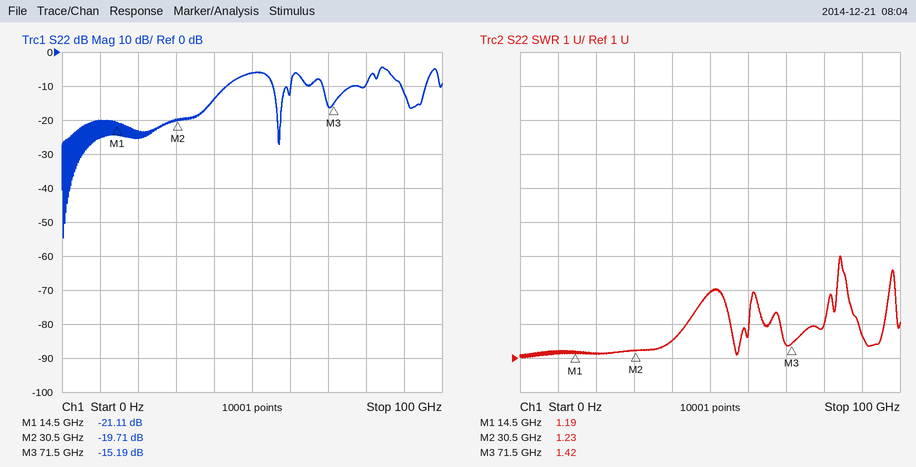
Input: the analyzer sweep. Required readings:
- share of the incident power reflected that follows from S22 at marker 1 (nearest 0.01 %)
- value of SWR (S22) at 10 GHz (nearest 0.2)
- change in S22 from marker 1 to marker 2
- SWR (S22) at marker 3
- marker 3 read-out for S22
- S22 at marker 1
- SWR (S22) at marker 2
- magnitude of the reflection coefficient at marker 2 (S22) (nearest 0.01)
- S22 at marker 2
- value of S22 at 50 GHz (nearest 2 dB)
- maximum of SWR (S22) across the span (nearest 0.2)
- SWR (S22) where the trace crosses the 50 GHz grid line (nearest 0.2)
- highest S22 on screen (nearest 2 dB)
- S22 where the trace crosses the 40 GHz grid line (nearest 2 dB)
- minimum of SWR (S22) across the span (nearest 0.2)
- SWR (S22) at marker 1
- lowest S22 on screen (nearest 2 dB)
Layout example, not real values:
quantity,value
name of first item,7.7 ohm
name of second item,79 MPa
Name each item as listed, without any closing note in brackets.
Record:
quantity,value
share of the incident power reflected that follows from S22 at marker 1,0.77 %
value of SWR (S22) at 10 GHz,1.2
change in S22 from marker 1 to marker 2,1.40 dB
SWR (S22) at marker 3,1.42
marker 3 read-out for S22,-15.19 dB
S22 at marker 1,-21.11 dB
SWR (S22) at marker 2,1.23
magnitude of the reflection coefficient at marker 2 (S22),0.10
S22 at marker 2,-19.71 dB
value of S22 at 50 GHz,-6 dB
maximum of SWR (S22) across the span,4.0
SWR (S22) where the trace crosses the 50 GHz grid line,3.0
highest S22 on screen,-4 dB
S22 where the trace crosses the 40 GHz grid line,-14 dB
minimum of SWR (S22) across the span,1.0
SWR (S22) at marker 1,1.19
lowest S22 on screen,-54 dB
